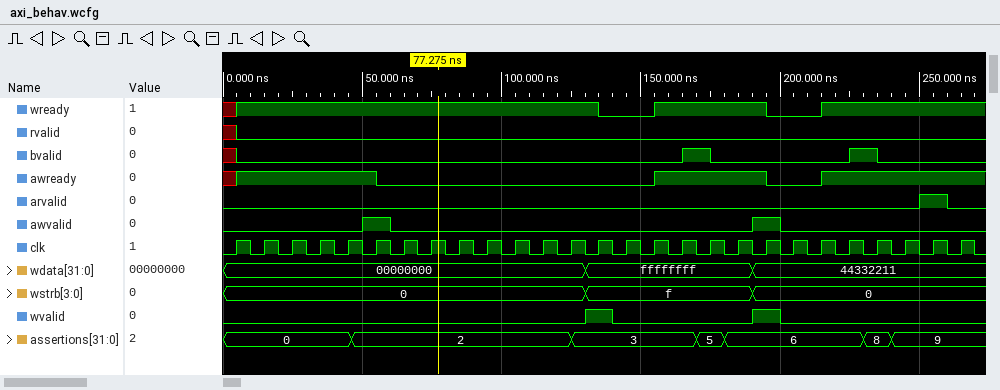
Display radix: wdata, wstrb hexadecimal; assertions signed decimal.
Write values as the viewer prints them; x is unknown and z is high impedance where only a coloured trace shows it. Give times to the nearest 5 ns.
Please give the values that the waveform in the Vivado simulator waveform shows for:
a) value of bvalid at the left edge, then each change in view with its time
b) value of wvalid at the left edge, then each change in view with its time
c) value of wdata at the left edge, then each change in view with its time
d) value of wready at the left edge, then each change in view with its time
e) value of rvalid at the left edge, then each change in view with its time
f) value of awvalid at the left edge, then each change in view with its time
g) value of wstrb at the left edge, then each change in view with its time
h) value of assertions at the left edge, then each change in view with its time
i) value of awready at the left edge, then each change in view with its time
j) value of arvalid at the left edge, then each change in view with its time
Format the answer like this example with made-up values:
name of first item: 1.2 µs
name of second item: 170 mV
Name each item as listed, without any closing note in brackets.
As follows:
value of bvalid at the left edge, then each change in view with its time: x, 0 at 5 ns, 1 at 165 ns, 0 at 175 ns, 1 at 225 ns, 0 at 235 ns
value of wvalid at the left edge, then each change in view with its time: 0, 1 at 130 ns, 0 at 140 ns, 1 at 190 ns, 0 at 200 ns
value of wdata at the left edge, then each change in view with its time: 00000000, ffffffff at 130 ns, 44332211 at 190 ns
value of wready at the left edge, then each change in view with its time: x, 1 at 5 ns, 0 at 135 ns, 1 at 155 ns, 0 at 195 ns, 1 at 215 ns
value of rvalid at the left edge, then each change in view with its time: x, 0 at 5 ns
value of awvalid at the left edge, then each change in view with its time: 0, 1 at 50 ns, 0 at 60 ns, 1 at 190 ns, 0 at 200 ns
value of wstrb at the left edge, then each change in view with its time: 0, f at 130 ns, 0 at 190 ns
value of assertions at the left edge, then each change in view with its time: 0, 2 at 45 ns, 3 at 125 ns, 5 at 170 ns, 6 at 180 ns, 8 at 230 ns, 9 at 240 ns
value of awready at the left edge, then each change in view with its time: x, 1 at 5 ns, 0 at 55 ns, 1 at 155 ns, 0 at 195 ns, 1 at 215 ns
value of arvalid at the left edge, then each change in view with its time: 0, 1 at 250 ns, 0 at 260 ns
